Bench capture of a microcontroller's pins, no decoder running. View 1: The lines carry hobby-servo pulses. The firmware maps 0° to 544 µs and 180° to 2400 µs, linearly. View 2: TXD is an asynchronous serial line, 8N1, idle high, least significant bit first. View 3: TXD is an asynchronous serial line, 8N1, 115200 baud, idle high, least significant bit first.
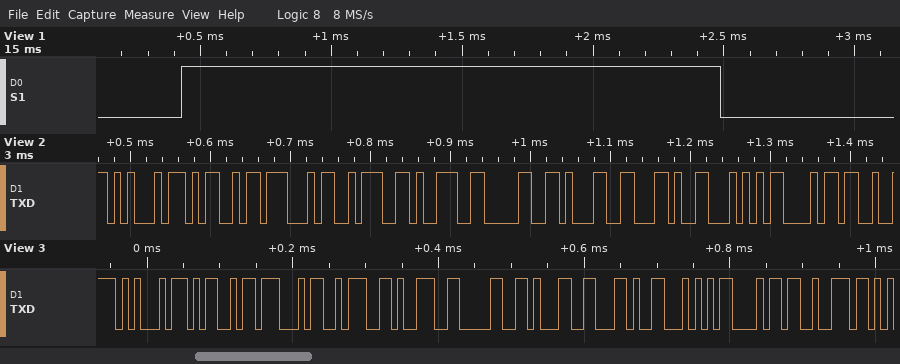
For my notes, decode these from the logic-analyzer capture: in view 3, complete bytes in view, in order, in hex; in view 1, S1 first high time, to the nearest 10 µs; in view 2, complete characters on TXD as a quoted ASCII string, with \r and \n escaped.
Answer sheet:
0x45 0x4D 0x47 0x3A 0x39 0x30 0x31 0x2C 0x54 0x68 0x72
2060 µs
"EMG:901,Th"
